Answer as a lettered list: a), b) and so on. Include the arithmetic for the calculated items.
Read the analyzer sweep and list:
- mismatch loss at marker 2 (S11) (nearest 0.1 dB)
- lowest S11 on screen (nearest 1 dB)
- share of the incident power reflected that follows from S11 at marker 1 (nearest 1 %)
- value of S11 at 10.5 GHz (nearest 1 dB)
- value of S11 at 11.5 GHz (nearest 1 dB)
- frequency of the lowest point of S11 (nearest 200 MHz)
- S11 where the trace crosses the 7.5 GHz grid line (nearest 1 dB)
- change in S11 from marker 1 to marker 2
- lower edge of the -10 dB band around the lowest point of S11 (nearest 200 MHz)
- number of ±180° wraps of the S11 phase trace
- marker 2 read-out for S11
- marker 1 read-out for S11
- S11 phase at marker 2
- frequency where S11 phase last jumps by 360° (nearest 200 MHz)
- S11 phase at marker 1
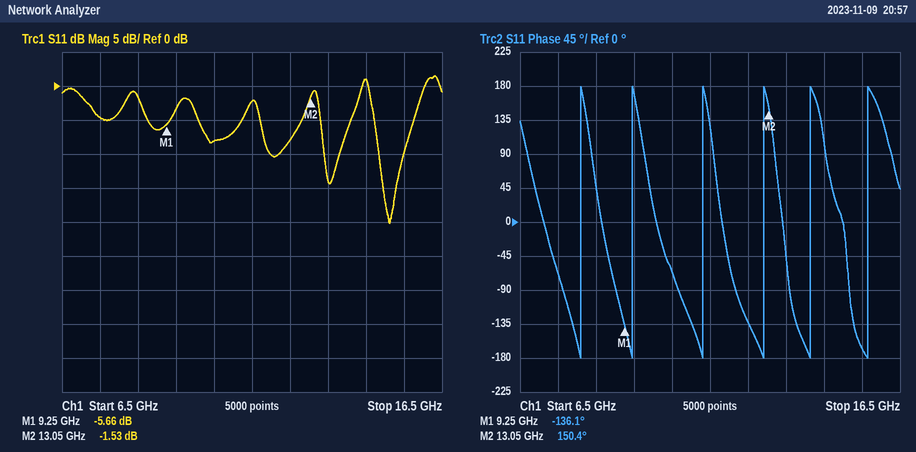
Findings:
a) −10 log10(1 − 10^(-1.53/10)) ≈ 5.3 dB
b) -20 dB
c) 10^(-5.66/10) ≈ 27 %
d) -8 dB
e) -2 dB
f) 15.2 GHz
g) -5 dB
h) -1.53 − (-5.66) = 4.13 dB
i) 14.8 GHz
j) 6
k) -1.53 dB
l) -5.66 dB
m) 150.4°
n) 15.6 GHz
o) -136.1°
